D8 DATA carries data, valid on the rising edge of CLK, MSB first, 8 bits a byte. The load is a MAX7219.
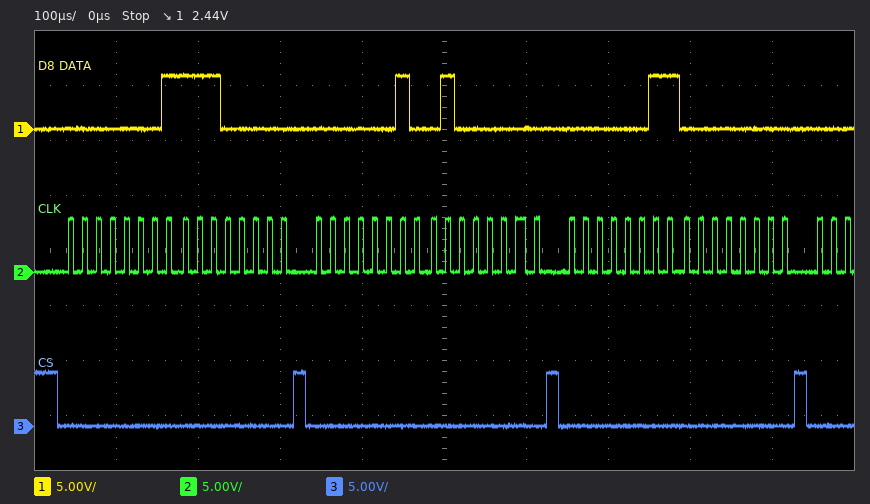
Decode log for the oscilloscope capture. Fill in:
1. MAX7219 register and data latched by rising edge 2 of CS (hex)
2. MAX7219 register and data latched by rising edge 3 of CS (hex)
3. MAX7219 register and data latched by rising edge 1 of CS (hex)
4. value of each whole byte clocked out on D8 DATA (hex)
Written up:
register 0x2, data 0x40
register 0x3, data 0x00
register 0x1, data 0xE0
01 E0 02 40 03 00
